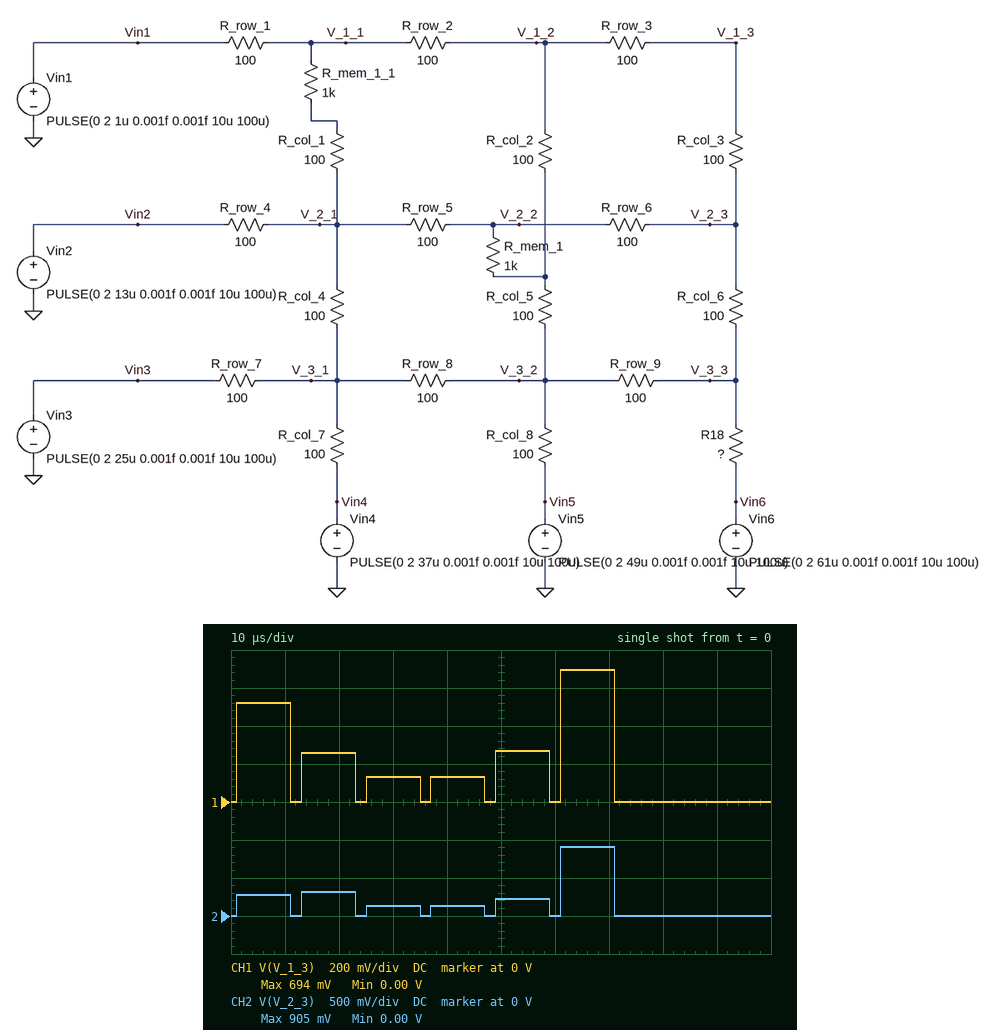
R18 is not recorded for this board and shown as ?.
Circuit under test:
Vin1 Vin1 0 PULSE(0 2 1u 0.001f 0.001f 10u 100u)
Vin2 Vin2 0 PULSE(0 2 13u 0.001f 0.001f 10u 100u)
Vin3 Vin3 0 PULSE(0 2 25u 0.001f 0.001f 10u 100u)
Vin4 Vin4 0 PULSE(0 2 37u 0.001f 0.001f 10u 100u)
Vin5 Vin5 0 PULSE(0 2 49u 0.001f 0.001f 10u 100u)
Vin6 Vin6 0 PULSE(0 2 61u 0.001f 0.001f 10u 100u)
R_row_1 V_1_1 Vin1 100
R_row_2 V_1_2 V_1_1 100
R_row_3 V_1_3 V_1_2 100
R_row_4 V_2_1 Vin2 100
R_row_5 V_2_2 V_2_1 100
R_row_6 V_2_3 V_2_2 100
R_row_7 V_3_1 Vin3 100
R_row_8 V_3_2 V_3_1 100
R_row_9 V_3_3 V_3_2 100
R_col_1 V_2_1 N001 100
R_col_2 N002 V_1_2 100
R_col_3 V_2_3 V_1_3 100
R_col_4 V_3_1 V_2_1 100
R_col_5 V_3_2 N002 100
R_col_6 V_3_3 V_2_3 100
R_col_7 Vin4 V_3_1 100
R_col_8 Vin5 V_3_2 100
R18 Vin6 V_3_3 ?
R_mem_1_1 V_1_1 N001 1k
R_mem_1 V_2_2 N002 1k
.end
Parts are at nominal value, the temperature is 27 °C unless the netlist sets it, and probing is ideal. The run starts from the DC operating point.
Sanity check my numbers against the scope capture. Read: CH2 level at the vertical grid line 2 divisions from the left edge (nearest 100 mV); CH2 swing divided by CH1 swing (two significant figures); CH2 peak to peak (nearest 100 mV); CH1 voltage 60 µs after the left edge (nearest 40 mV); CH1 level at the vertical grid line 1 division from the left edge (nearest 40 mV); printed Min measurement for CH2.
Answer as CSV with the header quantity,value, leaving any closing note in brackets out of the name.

quantity,value
CH2 level at the vertical grid line 2 divisions from the left edge,300 mV
CH2 swing divided by CH1 swing,1.3
CH2 peak to peak,900 mV
CH1 voltage 60 µs after the left edge,0 V
CH1 level at the vertical grid line 1 division from the left edge,520 mV
printed Min measurement for CH2,0.00 V
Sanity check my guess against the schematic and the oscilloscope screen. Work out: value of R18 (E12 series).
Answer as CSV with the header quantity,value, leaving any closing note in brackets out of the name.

quantity,value
value of R18,39 Ω
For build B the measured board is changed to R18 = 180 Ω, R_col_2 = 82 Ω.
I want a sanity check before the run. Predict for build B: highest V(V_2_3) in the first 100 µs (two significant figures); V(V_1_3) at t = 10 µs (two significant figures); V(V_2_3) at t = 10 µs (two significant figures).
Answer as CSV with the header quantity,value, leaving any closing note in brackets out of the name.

quantity,value
highest V(V_2_3) in the first 100 µs,450 mV
V(V_1_3) at t = 10 µs,570 mV
V(V_2_3) at t = 10 µs,350 mV
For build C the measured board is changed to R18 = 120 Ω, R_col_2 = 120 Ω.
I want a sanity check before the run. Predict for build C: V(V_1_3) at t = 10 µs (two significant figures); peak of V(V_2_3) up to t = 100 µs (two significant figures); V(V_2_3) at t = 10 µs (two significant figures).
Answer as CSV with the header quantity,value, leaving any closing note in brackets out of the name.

quantity,value
V(V_1_3) at t = 10 µs,580 mV
peak of V(V_2_3) up to t = 100 µs,570 mV
V(V_2_3) at t = 10 µs,340 mV
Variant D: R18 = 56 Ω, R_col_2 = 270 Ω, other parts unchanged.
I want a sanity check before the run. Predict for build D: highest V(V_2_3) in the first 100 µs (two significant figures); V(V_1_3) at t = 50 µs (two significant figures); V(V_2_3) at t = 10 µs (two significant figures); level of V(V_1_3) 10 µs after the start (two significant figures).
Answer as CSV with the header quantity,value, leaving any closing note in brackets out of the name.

quantity,value
highest V(V_2_3) in the first 100 µs,800 mV
V(V_1_3) at t = 50 µs,250 mV
V(V_2_3) at t = 10 µs,320 mV
level of V(V_1_3) 10 µs after the start,610 mV
